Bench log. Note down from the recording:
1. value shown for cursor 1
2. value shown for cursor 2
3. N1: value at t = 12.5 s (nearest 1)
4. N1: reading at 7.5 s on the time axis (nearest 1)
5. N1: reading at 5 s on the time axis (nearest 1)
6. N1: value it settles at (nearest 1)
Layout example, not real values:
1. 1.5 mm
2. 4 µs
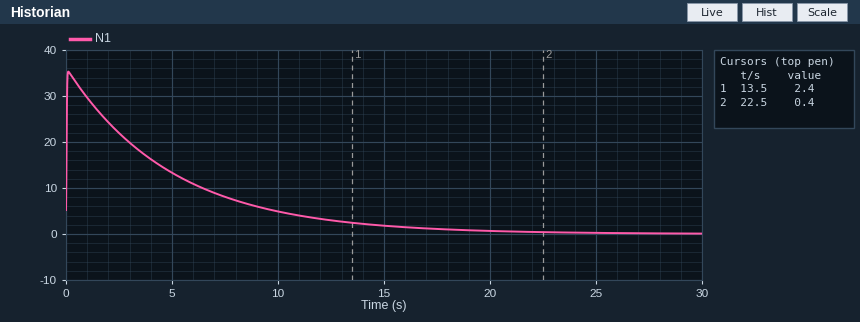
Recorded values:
1. 2.4
2. 0.4
3. 3
4. 8
5. 13
6. 0
